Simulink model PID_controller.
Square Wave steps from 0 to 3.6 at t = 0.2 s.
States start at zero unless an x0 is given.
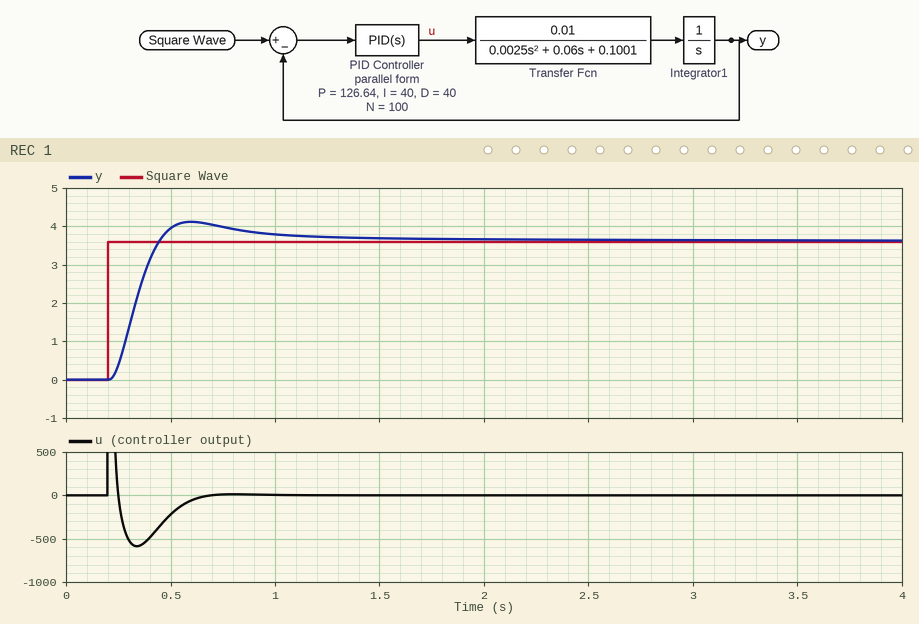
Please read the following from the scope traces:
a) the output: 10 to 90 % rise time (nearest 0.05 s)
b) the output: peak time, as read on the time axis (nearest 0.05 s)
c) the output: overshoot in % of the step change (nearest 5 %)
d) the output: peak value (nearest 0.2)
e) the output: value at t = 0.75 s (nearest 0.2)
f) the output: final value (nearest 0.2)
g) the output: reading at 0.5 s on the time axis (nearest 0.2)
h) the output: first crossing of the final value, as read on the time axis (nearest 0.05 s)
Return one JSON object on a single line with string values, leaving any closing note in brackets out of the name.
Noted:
{"the output: 10 to 90 % rise time": "0.15 s", "the output: peak time, as read on the time axis": "0.60 s", "the output: overshoot in % of the step change": "15 %", "the output: peak value": "4.2", "the output: value at t = 0.75 s": "4.0", "the output: final value": "3.6", "the output: reading at 0.5 s on the time axis": "4.0", "the output: first crossing of the final value, as read on the time axis": "0.45 s"}
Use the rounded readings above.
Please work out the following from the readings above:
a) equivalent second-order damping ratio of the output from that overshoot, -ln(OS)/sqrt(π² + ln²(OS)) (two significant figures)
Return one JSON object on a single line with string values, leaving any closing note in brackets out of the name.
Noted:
{"equivalent second-order damping ratio of the output from that overshoot, -ln(OS)/sqrt(π² + ln²(OS))": "0.52"}
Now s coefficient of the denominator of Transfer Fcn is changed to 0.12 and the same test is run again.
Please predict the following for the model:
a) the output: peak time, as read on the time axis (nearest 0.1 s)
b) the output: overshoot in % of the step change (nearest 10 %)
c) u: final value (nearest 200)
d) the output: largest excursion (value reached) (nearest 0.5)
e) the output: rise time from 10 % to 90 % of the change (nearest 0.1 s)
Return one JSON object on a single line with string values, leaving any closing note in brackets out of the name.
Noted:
{"the output: peak time, as read on the time axis": "1.0 s", "the output: overshoot in % of the step change": "20 %", "u: final value": "0", "the output: largest excursion (value reached)": "4.5", "the output: rise time from 10 % to 90 % of the change": "0.3 s"}
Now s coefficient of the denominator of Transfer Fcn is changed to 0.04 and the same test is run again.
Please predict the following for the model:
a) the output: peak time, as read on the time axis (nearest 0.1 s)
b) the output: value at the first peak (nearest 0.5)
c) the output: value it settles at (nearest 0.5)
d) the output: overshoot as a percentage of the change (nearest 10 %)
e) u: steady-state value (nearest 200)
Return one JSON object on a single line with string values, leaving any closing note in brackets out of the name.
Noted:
{"the output: peak time, as read on the time axis": "0.5 s", "the output: value at the first peak": "4.5", "the output: value it settles at": "3.5", "the output: overshoot as a percentage of the change": "20 %", "u: steady-state value": "0"}
